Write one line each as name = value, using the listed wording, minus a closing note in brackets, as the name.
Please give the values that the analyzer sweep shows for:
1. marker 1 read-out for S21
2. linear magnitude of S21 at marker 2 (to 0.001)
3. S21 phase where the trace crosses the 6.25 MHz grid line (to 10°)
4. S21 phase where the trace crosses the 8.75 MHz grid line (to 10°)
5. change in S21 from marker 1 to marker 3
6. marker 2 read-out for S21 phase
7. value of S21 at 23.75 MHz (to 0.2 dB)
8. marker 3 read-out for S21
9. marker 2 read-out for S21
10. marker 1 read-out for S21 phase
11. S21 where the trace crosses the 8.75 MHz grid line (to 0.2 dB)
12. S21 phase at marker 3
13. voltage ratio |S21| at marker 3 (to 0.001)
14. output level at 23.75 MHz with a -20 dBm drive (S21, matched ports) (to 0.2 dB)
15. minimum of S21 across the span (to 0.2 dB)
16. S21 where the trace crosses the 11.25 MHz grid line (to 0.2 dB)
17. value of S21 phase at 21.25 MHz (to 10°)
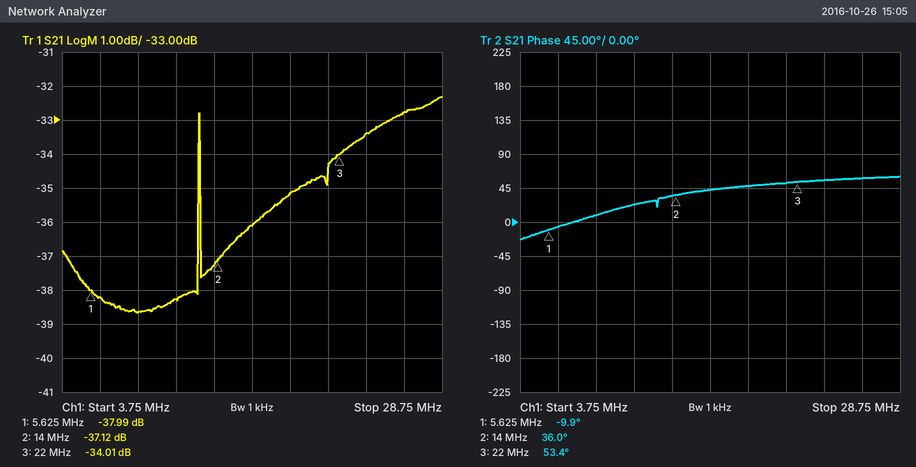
marker 1 read-out for S21 = -37.99 dB
linear magnitude of S21 at marker 2 = 0.014
S21 phase where the trace crosses the 6.25 MHz grid line = -10°
S21 phase where the trace crosses the 8.75 MHz grid line = 10°
change in S21 from marker 1 to marker 3 = 3.98 dB
marker 2 read-out for S21 phase = 36.0°
value of S21 at 23.75 MHz = -33.4 dB
marker 3 read-out for S21 = -34.01 dB
marker 2 read-out for S21 = -37.12 dB
marker 1 read-out for S21 phase = -9.9°
S21 where the trace crosses the 8.75 MHz grid line = -38.6 dB
S21 phase at marker 3 = 53.4°
voltage ratio |S21| at marker 3 = 0.020
output level at 23.75 MHz with a -20 dBm drive (S21, matched ports) = -53.4 dBm
minimum of S21 across the span = -38.6 dB
S21 where the trace crosses the 11.25 MHz grid line = -38.2 dB
value of S21 phase at 21.25 MHz = 50°
